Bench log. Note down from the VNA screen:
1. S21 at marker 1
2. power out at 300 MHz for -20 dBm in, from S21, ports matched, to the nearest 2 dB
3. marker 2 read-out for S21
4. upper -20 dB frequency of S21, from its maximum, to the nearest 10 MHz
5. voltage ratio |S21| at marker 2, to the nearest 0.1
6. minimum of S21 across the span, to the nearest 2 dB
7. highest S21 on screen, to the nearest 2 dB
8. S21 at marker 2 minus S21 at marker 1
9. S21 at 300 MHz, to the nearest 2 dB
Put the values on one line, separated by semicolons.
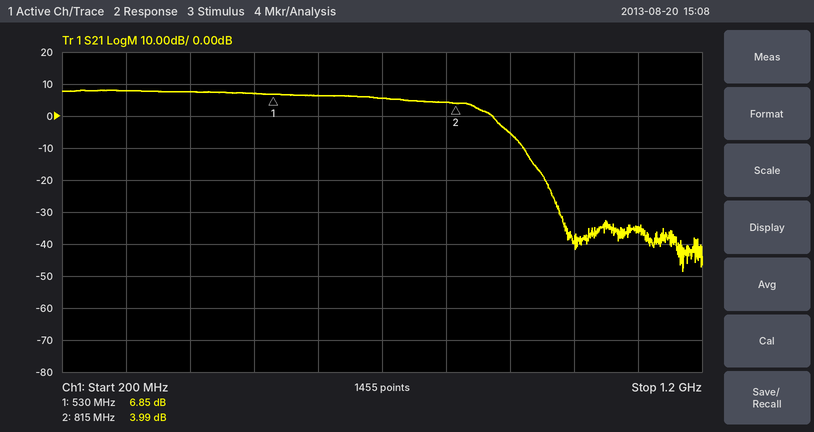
6.85 dB; -12 dBm; 3.99 dB; 930 MHz; 1.6; -48 dB; 8 dB; -2.86 dB; 8 dB
